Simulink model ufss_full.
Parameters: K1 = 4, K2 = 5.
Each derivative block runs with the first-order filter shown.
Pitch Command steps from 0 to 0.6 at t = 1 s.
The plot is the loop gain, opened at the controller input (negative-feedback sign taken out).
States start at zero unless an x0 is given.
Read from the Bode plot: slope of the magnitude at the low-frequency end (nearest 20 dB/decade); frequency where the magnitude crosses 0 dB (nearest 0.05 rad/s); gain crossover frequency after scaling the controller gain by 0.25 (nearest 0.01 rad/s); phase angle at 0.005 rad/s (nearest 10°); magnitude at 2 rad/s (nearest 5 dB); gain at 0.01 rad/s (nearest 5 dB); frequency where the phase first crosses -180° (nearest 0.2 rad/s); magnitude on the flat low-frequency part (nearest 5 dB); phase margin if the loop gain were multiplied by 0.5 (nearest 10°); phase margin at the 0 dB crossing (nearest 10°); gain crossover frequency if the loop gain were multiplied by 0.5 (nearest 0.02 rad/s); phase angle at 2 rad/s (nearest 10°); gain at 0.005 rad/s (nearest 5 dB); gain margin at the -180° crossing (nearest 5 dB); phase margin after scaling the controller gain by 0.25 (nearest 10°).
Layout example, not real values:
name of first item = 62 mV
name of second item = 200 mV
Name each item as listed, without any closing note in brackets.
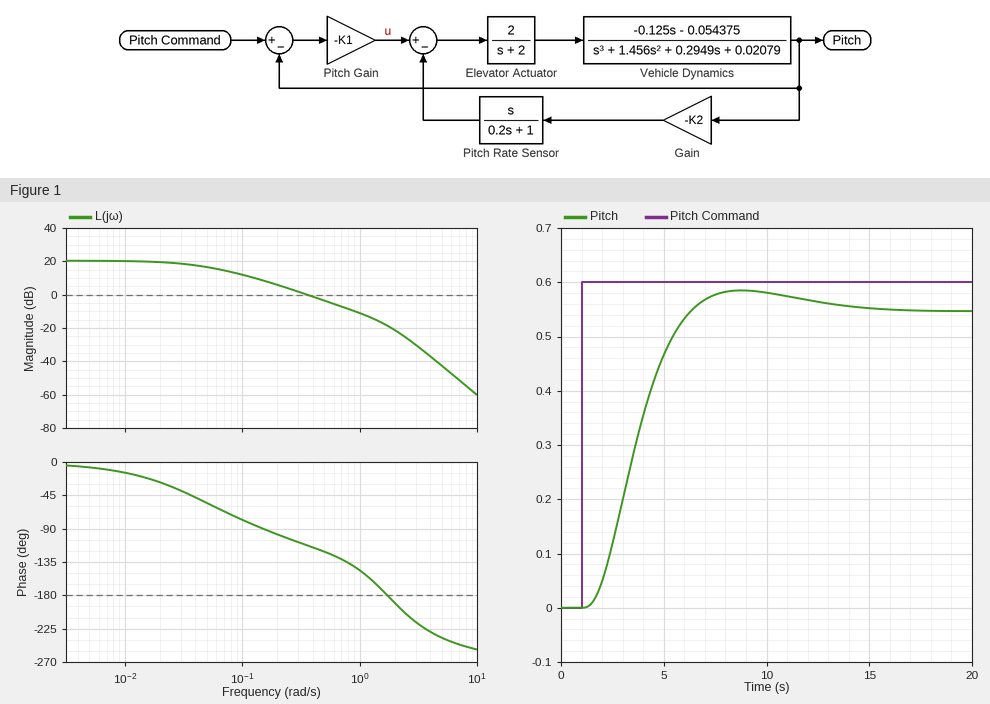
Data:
slope of the magnitude at the low-frequency end = 0 dB/decade
frequency where the magnitude crosses 0 dB = 0.35 rad/s
gain crossover frequency after scaling the controller gain by 0.25 = 0.10 rad/s
phase angle at 0.005 rad/s = -10°
magnitude at 2 rad/s = -20 dB
gain at 0.01 rad/s = 20 dB
frequency where the phase first crosses -180° = 1.8 rad/s
magnitude on the flat low-frequency part = 20 dB
phase margin if the loop gain were multiplied by 0.5 = 80°
phase margin at the 0 dB crossing = 70°
gain crossover frequency if the loop gain were multiplied by 0.5 = 0.20 rad/s
phase angle at 2 rad/s = -190°
gain at 0.005 rad/s = 20 dB
gain margin at the -180° crossing = 20 dB
phase margin after scaling the controller gain by 0.25 = 100°
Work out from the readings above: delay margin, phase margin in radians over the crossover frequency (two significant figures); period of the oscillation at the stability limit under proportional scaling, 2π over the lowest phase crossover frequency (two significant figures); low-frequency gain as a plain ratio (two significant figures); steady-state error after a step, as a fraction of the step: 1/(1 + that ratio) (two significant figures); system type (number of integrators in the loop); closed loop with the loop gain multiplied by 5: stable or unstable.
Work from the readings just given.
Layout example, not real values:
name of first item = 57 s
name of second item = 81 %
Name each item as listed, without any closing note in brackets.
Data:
delay margin, phase margin in radians over the crossover frequency = 3.5 s
period of the oscillation at the stability limit under proportional scaling, 2π over the lowest phase crossover frequency = 3.5 s
low-frequency gain as a plain ratio = 10
steady-state error after a step, as a fraction of the step: 1/(1 + that ratio) = 0.091
system type = 0
closed loop with the loop gain multiplied by 5: stable or unstable = stable
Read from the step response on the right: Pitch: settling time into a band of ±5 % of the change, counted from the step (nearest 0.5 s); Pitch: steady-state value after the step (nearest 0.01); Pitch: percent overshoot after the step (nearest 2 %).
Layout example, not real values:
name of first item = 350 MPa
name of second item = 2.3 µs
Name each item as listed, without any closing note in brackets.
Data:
Pitch: settling time into a band of ±5 % of the change, counted from the step = 10.0 s
Pitch: steady-state value after the step = 0.55
Pitch: percent overshoot after the step = 6 %
